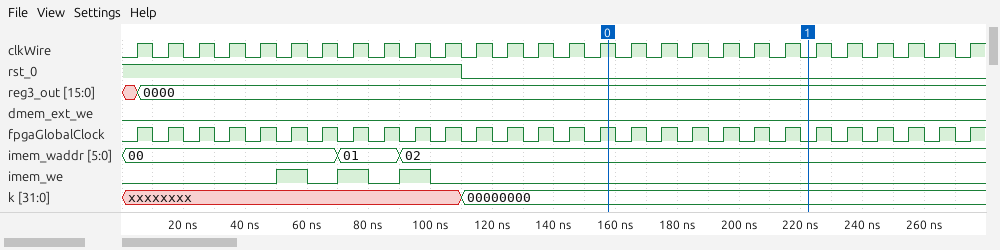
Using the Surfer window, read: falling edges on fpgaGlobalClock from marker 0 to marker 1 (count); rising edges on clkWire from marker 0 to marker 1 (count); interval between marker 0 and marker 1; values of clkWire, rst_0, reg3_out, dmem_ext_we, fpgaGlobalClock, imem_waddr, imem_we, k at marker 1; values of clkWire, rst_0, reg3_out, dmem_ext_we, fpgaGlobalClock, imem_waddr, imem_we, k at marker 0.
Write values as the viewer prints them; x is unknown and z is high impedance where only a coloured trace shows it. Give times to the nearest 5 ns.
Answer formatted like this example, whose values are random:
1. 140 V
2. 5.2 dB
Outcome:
1. 7
2. 6
3. 65 ns
4. clkWire=0, rst_0=0, reg3_out=0000, dmem_ext_we=0, fpgaGlobalClock=0, imem_waddr=02, imem_we=0, k=00000000
5. clkWire=1, rst_0=0, reg3_out=0000, dmem_ext_we=0, fpgaGlobalClock=1, imem_waddr=02, imem_we=0, k=00000000
